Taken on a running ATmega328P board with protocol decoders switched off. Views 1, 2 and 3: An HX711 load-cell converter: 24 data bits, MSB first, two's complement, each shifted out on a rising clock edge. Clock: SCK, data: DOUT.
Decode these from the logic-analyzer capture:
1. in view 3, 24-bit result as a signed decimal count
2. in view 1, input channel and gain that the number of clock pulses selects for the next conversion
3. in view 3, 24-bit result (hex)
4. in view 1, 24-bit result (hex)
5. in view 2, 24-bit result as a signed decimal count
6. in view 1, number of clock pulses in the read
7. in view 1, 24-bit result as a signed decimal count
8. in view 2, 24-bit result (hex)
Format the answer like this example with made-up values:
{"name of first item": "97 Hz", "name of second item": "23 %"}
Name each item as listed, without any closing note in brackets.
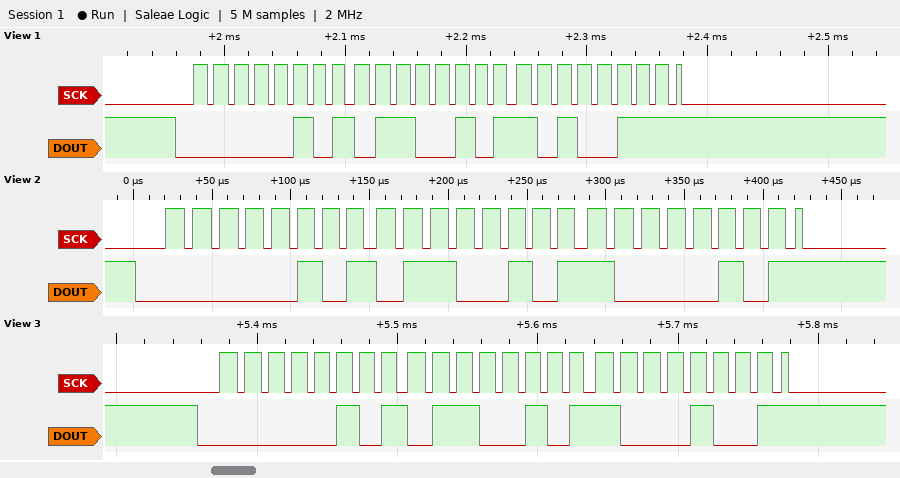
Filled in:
{"in view 3, 24-bit result as a signed decimal count": "353673", "in view 1, input channel and gain that the number of clock pulses selects for the next conversion": "channel A, gain 128", "in view 3, 24-bit result": "0x056589", "in view 1, 24-bit result": "0x0565A7", "in view 2, 24-bit result as a signed decimal count": "353669", "in view 1, number of clock pulses in the read": "25", "in view 1, 24-bit result as a signed decimal count": "353703", "in view 2, 24-bit result": "0x056585"}
